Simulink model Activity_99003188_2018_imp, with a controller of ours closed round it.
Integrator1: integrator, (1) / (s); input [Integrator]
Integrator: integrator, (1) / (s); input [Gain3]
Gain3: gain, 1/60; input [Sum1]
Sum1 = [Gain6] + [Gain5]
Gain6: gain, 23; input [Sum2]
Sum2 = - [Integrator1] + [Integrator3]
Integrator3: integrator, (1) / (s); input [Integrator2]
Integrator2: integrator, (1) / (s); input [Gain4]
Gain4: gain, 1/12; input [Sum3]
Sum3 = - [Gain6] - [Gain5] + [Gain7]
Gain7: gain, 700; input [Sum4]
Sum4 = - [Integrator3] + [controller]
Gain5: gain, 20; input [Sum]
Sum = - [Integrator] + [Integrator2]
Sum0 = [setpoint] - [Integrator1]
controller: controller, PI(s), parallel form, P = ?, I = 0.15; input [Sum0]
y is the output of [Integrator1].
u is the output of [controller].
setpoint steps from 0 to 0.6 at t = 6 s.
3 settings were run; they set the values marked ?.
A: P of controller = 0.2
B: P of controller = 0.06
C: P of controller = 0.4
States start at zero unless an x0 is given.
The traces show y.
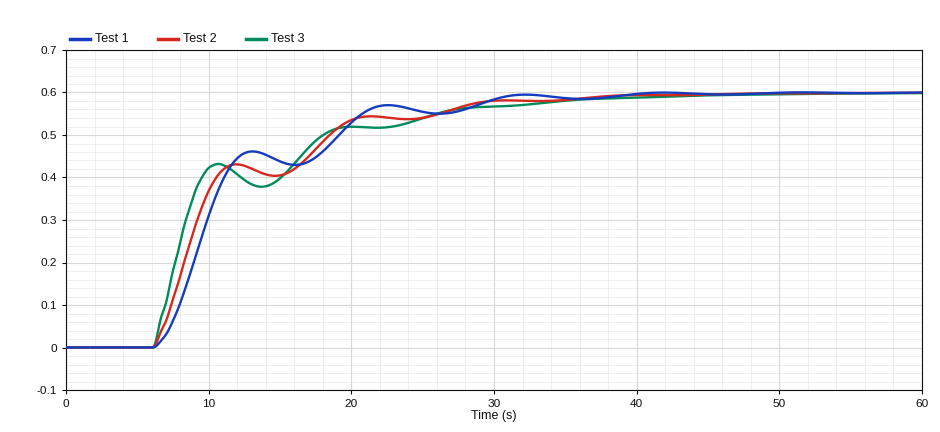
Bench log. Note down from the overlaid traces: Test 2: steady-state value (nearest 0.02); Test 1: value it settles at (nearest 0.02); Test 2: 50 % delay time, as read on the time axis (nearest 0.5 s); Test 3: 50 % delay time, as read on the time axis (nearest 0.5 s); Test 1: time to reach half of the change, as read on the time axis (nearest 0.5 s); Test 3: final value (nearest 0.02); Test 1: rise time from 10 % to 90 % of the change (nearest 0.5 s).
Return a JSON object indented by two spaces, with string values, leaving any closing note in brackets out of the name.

{
  "Test 2: steady-state value": "0.60",
  "Test 1: value it settles at": "0.60",
  "Test 2: 50 % delay time, as read on the time axis": "9.0 s",
  "Test 3: 50 % delay time, as read on the time axis": "8.5 s",
  "Test 1: time to reach half of the change, as read on the time axis": "10.0 s",
  "Test 3: final value": "0.60",
  "Test 1: rise time from 10 % to 90 % of the change": "13.0 s"
}
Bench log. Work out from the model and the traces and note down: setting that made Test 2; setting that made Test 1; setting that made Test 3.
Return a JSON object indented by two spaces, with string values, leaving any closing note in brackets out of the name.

{
  "setting that made Test 2": "A",
  "setting that made Test 1": "B",
  "setting that made Test 3": "C"
}
